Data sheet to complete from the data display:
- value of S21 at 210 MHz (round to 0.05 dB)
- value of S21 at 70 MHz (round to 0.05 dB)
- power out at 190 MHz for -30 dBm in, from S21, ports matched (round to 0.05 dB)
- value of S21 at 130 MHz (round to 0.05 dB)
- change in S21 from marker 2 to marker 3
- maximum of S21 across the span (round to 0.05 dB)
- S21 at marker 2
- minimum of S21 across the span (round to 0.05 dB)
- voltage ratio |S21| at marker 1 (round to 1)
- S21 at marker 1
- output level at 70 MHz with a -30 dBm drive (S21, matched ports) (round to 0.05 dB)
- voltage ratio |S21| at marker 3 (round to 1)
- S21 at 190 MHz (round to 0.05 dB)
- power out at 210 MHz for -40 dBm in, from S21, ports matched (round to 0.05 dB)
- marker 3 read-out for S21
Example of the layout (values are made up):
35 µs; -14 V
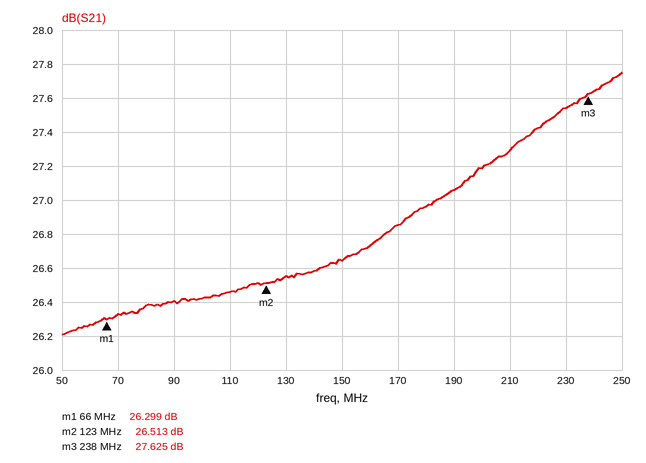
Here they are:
27.30 dB; 26.35 dB; -2.95 dBm; 26.55 dB; 1.112 dB; 27.75 dB; 26.513 dB; 26.20 dB; 21; 26.299 dB; -3.65 dBm; 24; 27.05 dB; -12.70 dBm; 27.625 dB
